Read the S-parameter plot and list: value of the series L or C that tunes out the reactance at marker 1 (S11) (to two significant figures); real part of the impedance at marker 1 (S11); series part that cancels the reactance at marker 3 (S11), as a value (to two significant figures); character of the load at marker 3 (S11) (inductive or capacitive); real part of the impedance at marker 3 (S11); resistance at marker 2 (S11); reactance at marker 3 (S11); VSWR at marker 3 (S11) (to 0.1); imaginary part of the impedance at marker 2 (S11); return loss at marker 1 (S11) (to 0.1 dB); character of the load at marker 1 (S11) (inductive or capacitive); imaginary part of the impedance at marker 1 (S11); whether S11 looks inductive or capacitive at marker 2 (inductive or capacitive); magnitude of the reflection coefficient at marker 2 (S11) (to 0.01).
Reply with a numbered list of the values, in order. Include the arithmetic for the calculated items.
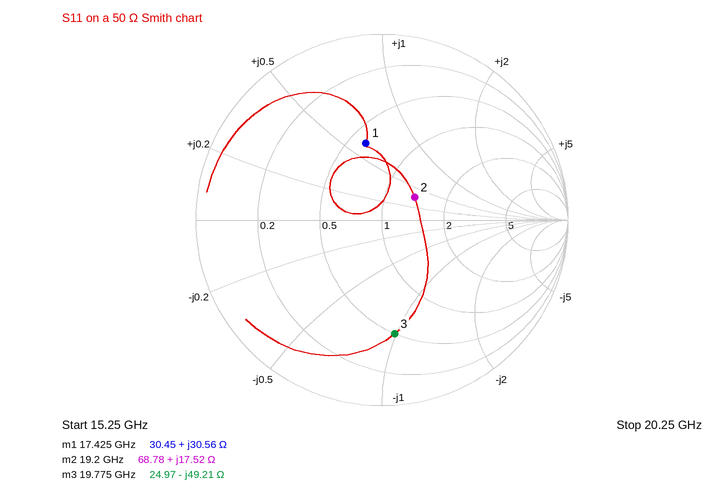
1. C = 1/(2π × 17.425 GHz × 30.56 Ω) ≈ 299 fF, so 300 fF to two significant figures
2. 30.45 Ω
3. L = 49.21 Ω/(2π × 19.775 GHz) ≈ 396 pH, so 400 pH to two significant figures
4. capacitive
5. 24.97 Ω
6. 68.78 Ω
7. -49.21 Ω
8. 4.2
9. +17.52 Ω
10. 7.5 dB
11. inductive
12. +30.56 Ω
13. inductive
14. 0.21
